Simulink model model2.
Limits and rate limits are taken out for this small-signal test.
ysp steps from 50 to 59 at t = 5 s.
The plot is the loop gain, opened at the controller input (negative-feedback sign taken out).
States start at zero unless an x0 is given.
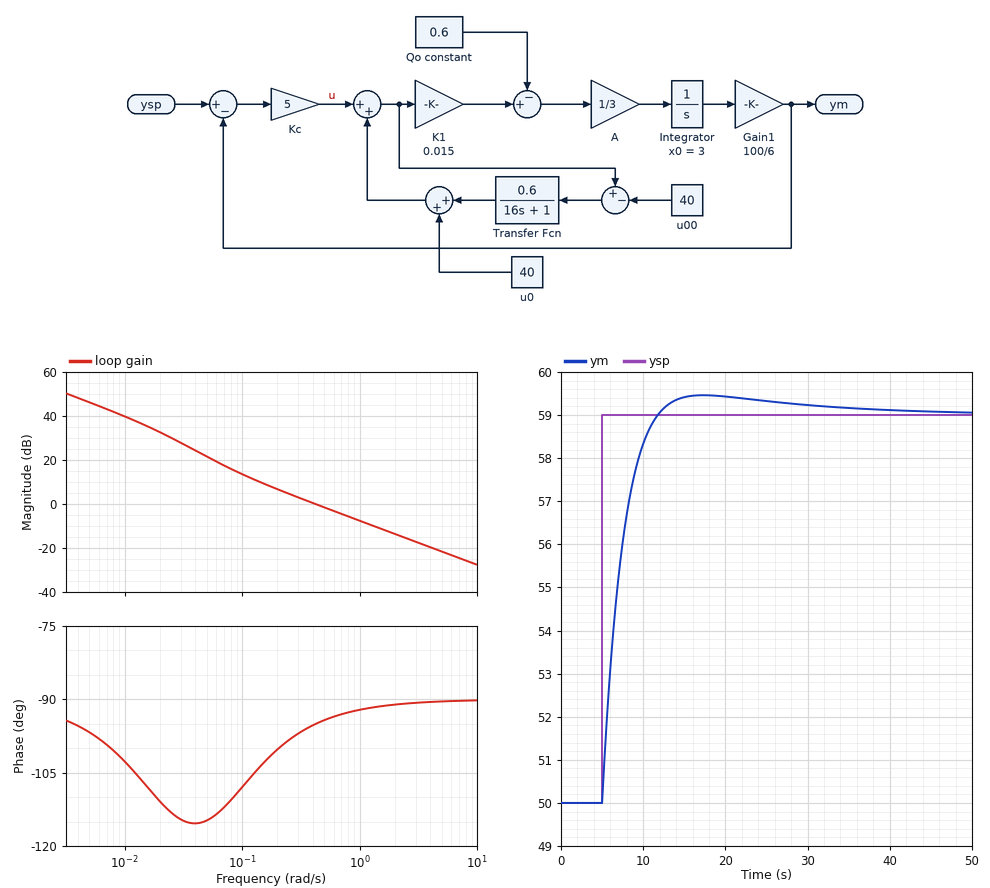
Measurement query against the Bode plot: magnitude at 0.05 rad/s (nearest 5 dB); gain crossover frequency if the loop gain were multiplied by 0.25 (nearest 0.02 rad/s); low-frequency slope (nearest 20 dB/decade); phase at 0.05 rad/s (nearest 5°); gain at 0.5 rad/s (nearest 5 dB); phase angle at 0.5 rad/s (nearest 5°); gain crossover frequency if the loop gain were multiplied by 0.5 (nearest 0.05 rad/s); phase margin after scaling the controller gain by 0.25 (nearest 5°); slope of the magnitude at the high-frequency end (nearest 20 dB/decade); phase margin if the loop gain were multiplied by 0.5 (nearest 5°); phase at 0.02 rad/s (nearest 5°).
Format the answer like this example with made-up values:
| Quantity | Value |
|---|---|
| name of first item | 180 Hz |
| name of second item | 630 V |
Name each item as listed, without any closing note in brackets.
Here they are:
| Quantity | Value |
|---|---|
| magnitude at 0.05 rad/s | 20 dB |
| gain crossover frequency if the loop gain were multiplied by 0.25 | 0.12 rad/s |
| low-frequency slope | -20 dB/decade |
| phase at 0.05 rad/s | -115° |
| gain at 0.5 rad/s | 0 dB |
| phase angle at 0.5 rad/s | -95° |
| gain crossover frequency if the loop gain were multiplied by 0.5 | 0.20 rad/s |
| phase margin after scaling the controller gain by 0.25 | 75° |
| slope of the magnitude at the high-frequency end | -20 dB/decade |
| phase margin if the loop gain were multiplied by 0.5 | 80° |
| phase at 0.02 rad/s | -110° |
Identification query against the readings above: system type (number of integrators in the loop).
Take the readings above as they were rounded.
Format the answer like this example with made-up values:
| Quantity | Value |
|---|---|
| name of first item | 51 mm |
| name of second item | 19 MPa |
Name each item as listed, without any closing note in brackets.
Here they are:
| Quantity | Value |
|---|---|
| system type | 1 |
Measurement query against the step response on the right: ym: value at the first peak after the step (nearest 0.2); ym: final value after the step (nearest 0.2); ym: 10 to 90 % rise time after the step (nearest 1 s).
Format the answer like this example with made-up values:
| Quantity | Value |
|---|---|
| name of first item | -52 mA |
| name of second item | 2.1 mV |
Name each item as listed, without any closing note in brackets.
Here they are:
| Quantity | Value |
|---|---|
| ym: value at the first peak after the step | 59.4 |
| ym: final value after the step | 59.0 |
| ym: 10 to 90 % rise time after the step | 4 s |
